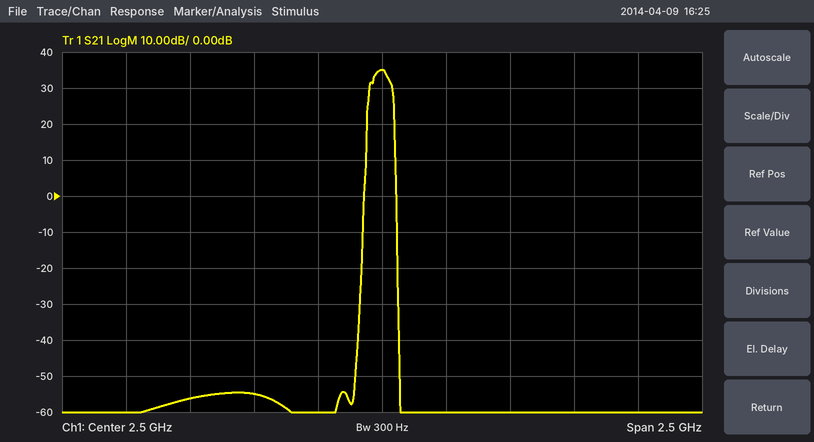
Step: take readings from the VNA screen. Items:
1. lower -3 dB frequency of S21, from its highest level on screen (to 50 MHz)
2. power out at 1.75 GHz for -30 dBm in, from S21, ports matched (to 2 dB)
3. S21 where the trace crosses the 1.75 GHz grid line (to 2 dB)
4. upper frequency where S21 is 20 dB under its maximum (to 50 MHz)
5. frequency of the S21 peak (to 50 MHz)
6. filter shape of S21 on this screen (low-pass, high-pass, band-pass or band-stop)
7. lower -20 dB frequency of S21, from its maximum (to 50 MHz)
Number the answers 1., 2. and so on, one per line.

1. 2.45 GHz
2. -86 dBm
3. -56 dB
4. 2.55 GHz
5. 2.50 GHz
6. band-pass
7. 2.45 GHz
